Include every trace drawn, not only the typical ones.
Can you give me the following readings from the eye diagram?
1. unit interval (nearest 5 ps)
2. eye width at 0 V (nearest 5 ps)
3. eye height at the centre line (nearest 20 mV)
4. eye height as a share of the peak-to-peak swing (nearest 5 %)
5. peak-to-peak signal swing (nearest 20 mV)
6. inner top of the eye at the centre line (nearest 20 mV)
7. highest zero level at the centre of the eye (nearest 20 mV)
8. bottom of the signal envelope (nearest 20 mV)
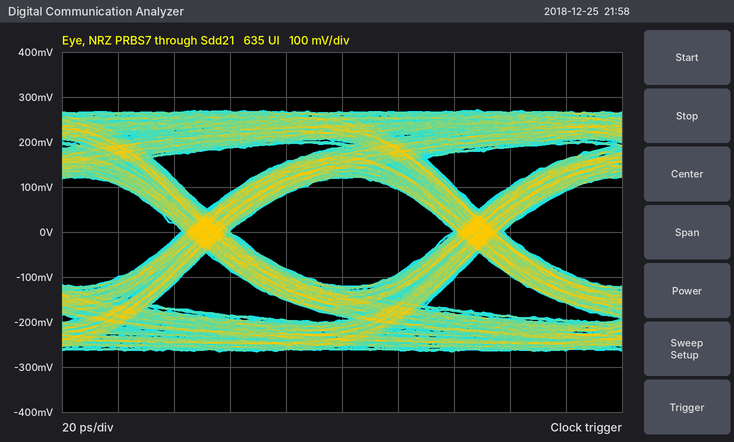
95 ps
80 ps
240 mV
45 %
540 mV
120 mV
-120 mV
-260 mV
